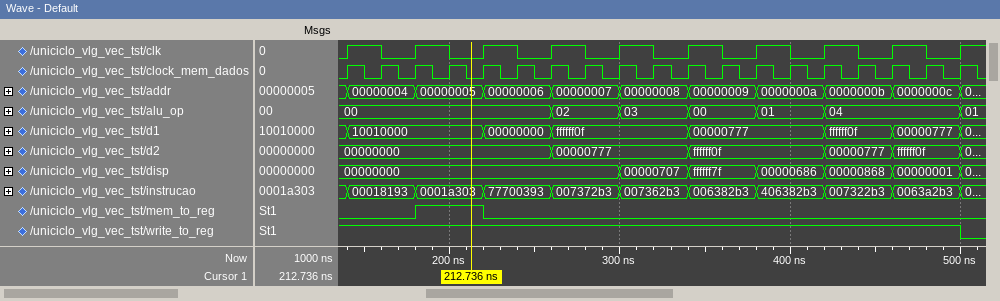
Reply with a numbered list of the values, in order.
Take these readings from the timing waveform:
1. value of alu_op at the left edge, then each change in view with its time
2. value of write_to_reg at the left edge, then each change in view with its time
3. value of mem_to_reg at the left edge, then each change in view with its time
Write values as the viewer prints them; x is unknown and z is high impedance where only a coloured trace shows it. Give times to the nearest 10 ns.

1. 00, 02 at 260 ns, 03 at 300 ns, 00 at 340 ns, 01 at 380 ns, 04 at 420 ns, 01 at 500 ns
2. 1, 0 at 500 ns
3. 0, 1 at 180 ns, 0 at 220 ns
